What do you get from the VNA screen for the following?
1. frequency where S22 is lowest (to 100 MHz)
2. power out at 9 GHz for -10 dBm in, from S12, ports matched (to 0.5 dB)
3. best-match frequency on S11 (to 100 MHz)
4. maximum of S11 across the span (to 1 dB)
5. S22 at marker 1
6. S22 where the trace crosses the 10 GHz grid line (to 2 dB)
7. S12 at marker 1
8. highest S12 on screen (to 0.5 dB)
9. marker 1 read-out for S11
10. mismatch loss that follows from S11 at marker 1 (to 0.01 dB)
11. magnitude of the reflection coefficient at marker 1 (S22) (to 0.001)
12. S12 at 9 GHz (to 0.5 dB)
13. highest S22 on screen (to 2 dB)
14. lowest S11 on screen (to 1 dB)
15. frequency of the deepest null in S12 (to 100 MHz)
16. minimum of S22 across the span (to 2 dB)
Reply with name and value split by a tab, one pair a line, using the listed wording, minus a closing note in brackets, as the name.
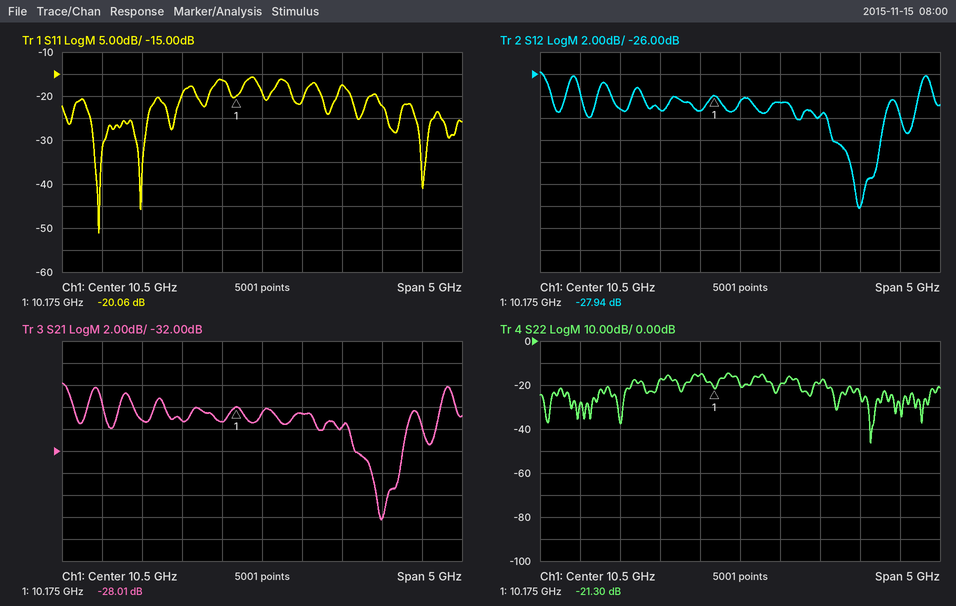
frequency where S22 is lowest	12.1 GHz
power out at 9 GHz for -10 dBm in, from S12, ports matched	-39.0 dBm
best-match frequency on S11	8.5 GHz
maximum of S11 across the span	-16 dB
S22 at marker 1	-21.30 dB
S22 where the trace crosses the 10 GHz grid line	-16 dB
S12 at marker 1	-27.94 dB
highest S12 on screen	-26.0 dB
marker 1 read-out for S11	-20.06 dB
mismatch loss that follows from S11 at marker 1	0.04 dB
magnitude of the reflection coefficient at marker 1 (S22)	0.086
S12 at 9 GHz	-29.0 dB
highest S22 on screen	-14 dB
lowest S11 on screen	-51 dB
frequency of the deepest null in S12	12.0 GHz
minimum of S22 across the span	-46 dB
